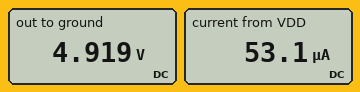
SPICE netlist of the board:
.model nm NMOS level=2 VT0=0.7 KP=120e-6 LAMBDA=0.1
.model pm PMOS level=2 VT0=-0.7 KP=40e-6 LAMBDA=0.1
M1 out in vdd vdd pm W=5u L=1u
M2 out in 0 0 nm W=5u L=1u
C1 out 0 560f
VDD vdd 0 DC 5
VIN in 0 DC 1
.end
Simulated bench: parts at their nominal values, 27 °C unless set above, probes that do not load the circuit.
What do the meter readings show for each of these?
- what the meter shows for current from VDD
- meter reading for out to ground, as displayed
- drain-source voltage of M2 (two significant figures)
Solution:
53.1 µA
4.919 V
4.9 V
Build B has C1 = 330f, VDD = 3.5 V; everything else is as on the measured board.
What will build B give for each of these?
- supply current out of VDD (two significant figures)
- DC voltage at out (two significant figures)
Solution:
41 µA
3.4 V
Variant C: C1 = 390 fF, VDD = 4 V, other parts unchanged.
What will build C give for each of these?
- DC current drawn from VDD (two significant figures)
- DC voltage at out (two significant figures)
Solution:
44 µA
3.9 V
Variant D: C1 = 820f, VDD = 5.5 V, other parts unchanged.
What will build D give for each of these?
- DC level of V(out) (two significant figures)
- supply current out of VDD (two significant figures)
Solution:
5.4 V
59 µA
